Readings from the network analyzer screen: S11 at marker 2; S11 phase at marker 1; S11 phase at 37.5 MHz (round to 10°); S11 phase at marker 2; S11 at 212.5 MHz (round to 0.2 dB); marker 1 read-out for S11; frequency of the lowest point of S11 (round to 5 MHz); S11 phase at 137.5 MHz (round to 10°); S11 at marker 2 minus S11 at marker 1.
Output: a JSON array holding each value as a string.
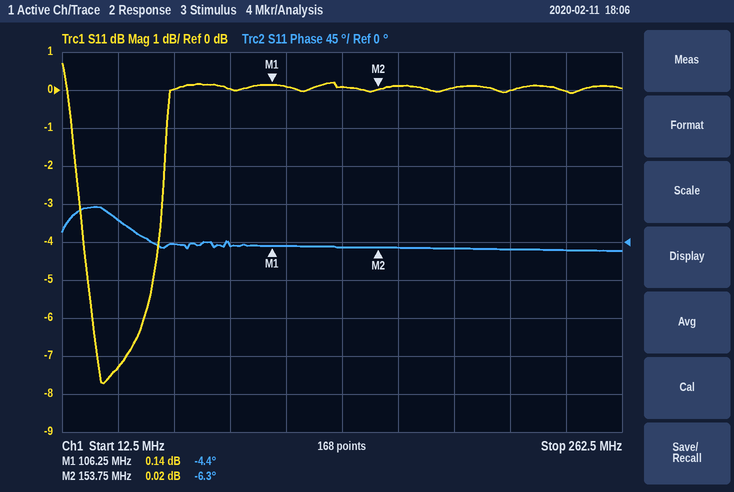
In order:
["0.02 dB", "-4.4°", "30°", "-6.3°", "0.0 dB", "0.14 dB", "30 MHz", "-10°", "-0.12 dB"]
